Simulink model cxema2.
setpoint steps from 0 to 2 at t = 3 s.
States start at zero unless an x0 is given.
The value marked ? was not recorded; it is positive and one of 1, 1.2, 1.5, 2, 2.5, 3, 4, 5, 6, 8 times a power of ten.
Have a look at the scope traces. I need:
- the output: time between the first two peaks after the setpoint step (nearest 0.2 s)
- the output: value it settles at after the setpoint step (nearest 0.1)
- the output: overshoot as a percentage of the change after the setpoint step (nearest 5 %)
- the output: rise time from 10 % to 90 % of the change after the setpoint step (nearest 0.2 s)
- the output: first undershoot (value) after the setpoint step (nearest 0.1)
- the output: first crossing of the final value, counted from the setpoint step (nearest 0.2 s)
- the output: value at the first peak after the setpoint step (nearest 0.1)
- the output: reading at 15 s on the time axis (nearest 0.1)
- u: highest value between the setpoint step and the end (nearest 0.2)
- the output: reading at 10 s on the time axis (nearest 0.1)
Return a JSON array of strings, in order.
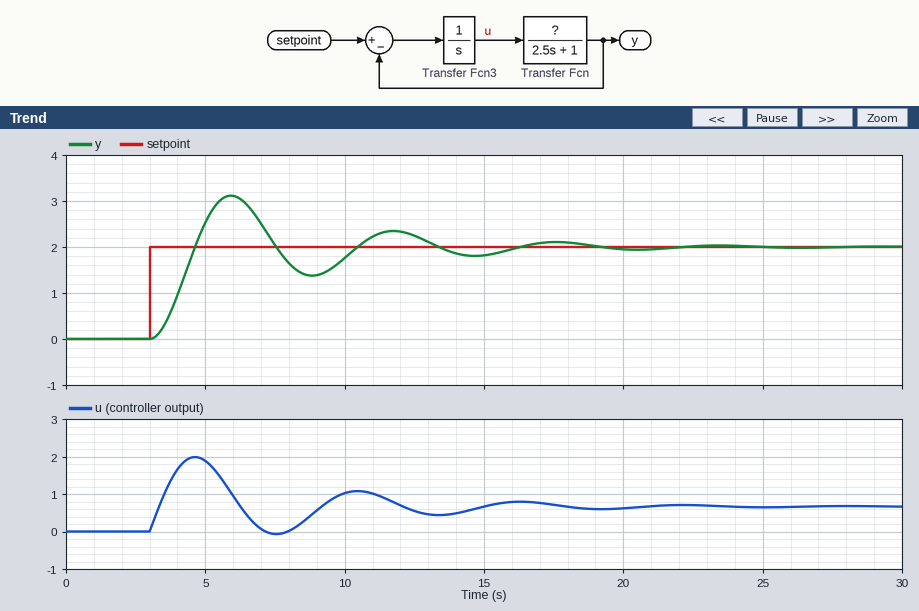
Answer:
["5.8 s", "2.0", "55 %", "1.0 s", "1.4", "1.6 s", "3.1", "1.8", "2.0", "1.8"]
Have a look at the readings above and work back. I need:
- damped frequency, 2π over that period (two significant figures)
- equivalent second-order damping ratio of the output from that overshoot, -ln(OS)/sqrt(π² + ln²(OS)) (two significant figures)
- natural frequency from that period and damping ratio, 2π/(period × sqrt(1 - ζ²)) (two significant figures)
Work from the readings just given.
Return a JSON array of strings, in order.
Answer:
["1.1 rad/s", "0.19", "1.1 rad/s"]
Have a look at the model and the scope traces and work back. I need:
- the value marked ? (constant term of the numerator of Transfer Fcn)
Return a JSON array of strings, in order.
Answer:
["3"]
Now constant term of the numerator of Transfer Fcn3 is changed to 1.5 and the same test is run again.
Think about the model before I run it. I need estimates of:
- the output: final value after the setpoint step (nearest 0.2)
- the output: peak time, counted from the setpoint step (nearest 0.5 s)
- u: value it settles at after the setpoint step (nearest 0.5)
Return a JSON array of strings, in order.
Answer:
["2.0", "2.5 s", "0.5"]
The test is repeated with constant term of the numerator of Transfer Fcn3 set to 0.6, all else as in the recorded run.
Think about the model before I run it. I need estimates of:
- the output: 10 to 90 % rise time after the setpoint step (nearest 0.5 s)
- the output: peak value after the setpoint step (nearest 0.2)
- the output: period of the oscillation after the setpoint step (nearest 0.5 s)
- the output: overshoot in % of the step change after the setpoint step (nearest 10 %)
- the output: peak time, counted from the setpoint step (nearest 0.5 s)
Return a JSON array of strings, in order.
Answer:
["1.5 s", "3.0", "7.5 s", "50 %", "4.0 s"]
